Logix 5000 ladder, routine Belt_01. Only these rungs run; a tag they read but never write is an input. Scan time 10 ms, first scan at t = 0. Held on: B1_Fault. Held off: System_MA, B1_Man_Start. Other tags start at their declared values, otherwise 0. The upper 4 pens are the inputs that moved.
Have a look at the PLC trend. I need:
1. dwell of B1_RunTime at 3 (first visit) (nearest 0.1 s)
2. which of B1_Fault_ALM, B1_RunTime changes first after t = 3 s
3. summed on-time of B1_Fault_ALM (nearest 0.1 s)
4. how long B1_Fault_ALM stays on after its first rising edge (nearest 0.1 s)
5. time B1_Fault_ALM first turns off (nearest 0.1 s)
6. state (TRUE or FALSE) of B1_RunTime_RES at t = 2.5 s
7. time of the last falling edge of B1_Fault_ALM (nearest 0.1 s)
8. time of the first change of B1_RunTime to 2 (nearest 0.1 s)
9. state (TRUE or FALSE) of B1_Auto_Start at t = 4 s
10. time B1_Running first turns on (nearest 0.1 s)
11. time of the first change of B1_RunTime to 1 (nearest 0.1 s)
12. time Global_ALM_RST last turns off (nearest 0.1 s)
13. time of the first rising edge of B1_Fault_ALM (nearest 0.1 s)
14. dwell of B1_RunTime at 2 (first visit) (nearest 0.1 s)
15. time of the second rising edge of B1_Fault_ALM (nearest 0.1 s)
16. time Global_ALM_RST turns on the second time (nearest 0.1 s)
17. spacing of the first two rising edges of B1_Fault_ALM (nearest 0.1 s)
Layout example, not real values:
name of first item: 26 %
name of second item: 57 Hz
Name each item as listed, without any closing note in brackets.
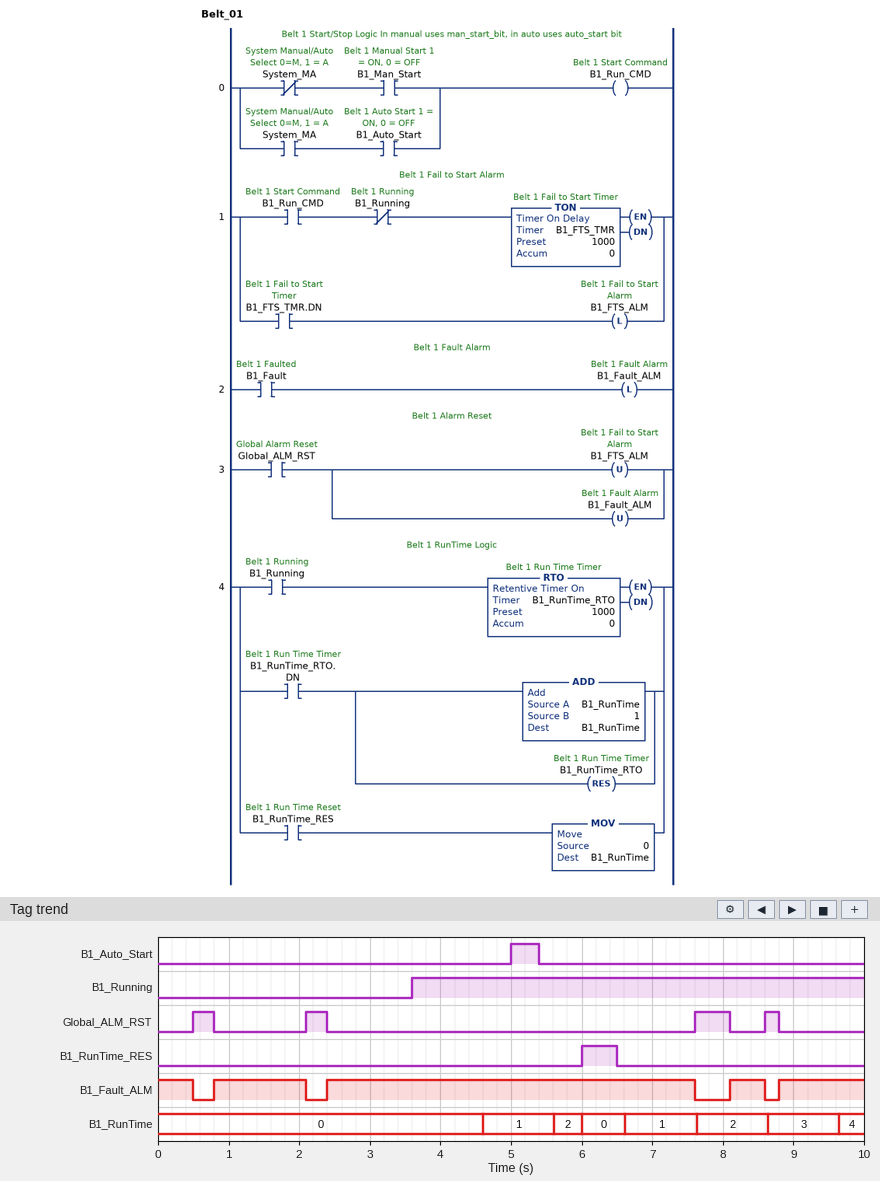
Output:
dwell of B1_RunTime at 3 (first visit): 1.0 s
which of B1_Fault_ALM, B1_RunTime changes first after t = 3 s: B1_RunTime
summed on-time of B1_Fault_ALM: 8.7 s
how long B1_Fault_ALM stays on after its first rising edge: 1.3 s
time B1_Fault_ALM first turns off: 0.5 s
state (TRUE or FALSE) of B1_RunTime_RES at t = 2.5 s: FALSE
time of the last falling edge of B1_Fault_ALM: 8.6 s
time of the first change of B1_RunTime to 2: 5.6 s
state (TRUE or FALSE) of B1_Auto_Start at t = 4 s: FALSE
time B1_Running first turns on: 3.6 s
time of the first change of B1_RunTime to 1: 4.6 s
time Global_ALM_RST last turns off: 8.8 s
time of the first rising edge of B1_Fault_ALM: 0.8 s
dwell of B1_RunTime at 2 (first visit): 0.4 s
time of the second rising edge of B1_Fault_ALM: 2.4 s
time Global_ALM_RST turns on the second time: 2.1 s
spacing of the first two rising edges of B1_Fault_ALM: 1.6 s
